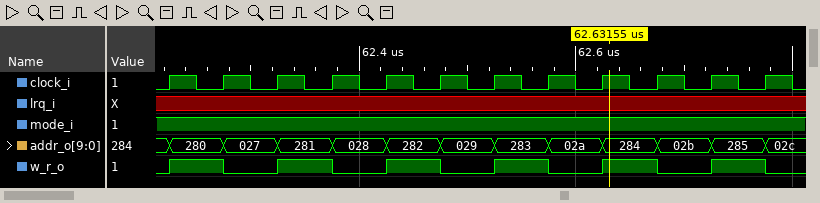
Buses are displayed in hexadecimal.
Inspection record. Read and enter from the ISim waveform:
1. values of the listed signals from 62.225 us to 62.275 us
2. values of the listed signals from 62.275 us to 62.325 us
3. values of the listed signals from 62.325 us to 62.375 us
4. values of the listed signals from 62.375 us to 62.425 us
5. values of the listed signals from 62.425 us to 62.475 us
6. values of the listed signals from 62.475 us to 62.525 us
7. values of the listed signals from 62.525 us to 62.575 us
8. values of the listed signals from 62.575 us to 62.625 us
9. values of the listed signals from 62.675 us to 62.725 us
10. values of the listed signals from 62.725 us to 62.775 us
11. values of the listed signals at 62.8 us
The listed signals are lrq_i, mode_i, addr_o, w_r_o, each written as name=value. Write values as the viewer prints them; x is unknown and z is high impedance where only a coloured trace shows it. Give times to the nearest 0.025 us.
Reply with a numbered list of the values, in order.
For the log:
1. lrq_i=x, mode_i=1, addr_o=280, w_r_o=1
2. lrq_i=x, mode_i=1, addr_o=027, w_r_o=0
3. lrq_i=x, mode_i=1, addr_o=281, w_r_o=1
4. lrq_i=x, mode_i=1, addr_o=028, w_r_o=0
5. lrq_i=x, mode_i=1, addr_o=282, w_r_o=1
6. lrq_i=x, mode_i=1, addr_o=029, w_r_o=0
7. lrq_i=x, mode_i=1, addr_o=283, w_r_o=1
8. lrq_i=x, mode_i=1, addr_o=02a, w_r_o=0
9. lrq_i=x, mode_i=1, addr_o=02b, w_r_o=0
10. lrq_i=x, mode_i=1, addr_o=285, w_r_o=1
11. lrq_i=x, mode_i=1, addr_o=02c, w_r_o=0
